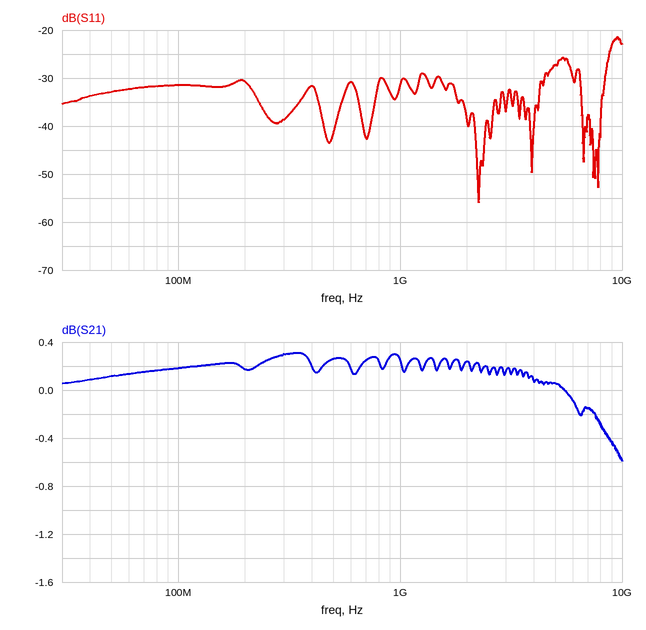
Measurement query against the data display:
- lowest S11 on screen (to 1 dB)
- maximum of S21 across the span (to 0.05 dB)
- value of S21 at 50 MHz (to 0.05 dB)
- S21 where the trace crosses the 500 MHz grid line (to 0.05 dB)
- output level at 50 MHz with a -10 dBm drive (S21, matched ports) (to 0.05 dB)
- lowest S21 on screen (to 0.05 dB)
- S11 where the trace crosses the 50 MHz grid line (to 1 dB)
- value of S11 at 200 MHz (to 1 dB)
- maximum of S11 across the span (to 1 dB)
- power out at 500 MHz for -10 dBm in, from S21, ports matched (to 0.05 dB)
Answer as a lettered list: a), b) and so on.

a) -56 dB
b) 0.30 dB
c) 0.10 dB
d) 0.25 dB
e) -9.90 dBm
f) -0.60 dB
g) -33 dB
h) -31 dB
i) -21 dB
j) -9.75 dBm
